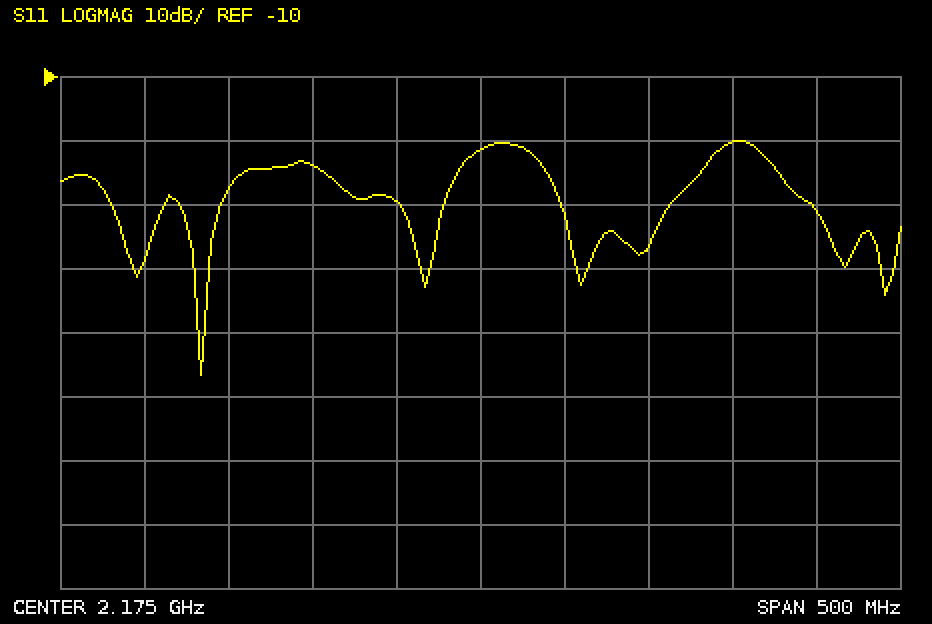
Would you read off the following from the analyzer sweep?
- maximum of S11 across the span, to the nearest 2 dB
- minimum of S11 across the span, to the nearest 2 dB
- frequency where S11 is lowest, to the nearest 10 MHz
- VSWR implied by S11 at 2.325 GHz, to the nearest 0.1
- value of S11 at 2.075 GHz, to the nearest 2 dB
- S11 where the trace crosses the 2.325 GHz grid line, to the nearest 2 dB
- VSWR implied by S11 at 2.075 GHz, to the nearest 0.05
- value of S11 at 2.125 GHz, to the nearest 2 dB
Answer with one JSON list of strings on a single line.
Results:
["-20 dB", "-56 dB", "2.01 GHz", "1.2", "-24 dB", "-20 dB", "1.15", "-30 dB"]
